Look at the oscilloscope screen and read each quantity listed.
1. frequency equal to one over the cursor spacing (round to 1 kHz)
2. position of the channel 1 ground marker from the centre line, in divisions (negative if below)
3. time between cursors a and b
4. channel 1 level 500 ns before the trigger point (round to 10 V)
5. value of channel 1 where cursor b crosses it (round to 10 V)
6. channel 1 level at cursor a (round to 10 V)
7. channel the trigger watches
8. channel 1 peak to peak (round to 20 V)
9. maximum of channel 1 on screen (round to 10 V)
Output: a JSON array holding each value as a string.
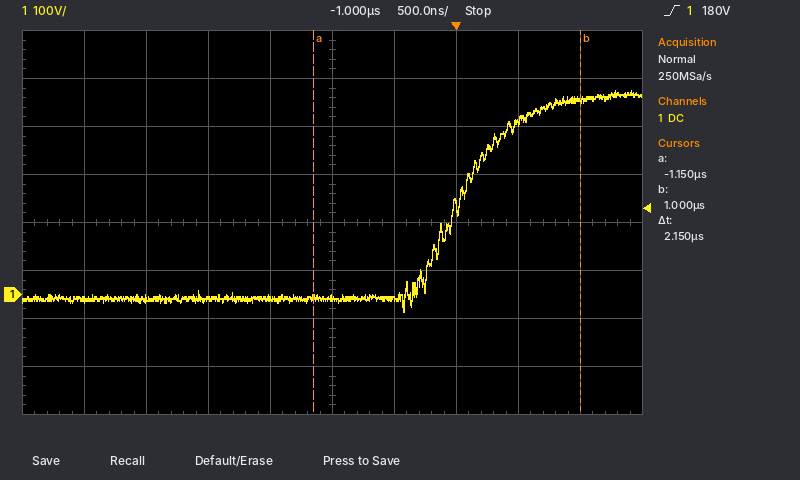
["465 kHz", "-1.5 div", "2.15 µs", "-10 V", "410 V", "-10 V", "channel 1", "460 V", "420 V"]
